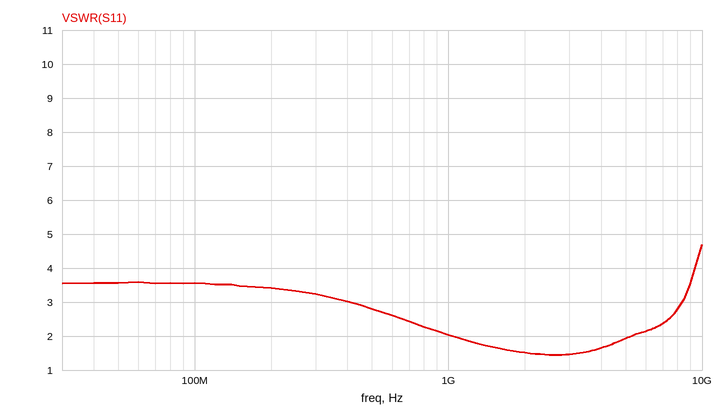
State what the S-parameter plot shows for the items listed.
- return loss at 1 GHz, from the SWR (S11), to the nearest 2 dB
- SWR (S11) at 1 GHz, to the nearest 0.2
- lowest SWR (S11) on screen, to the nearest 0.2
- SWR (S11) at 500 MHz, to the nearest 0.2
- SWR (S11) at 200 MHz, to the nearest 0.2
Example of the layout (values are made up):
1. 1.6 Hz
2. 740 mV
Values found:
1. 10 dB
2. 2.0
3. 1.4
4. 2.8
5. 3.4
